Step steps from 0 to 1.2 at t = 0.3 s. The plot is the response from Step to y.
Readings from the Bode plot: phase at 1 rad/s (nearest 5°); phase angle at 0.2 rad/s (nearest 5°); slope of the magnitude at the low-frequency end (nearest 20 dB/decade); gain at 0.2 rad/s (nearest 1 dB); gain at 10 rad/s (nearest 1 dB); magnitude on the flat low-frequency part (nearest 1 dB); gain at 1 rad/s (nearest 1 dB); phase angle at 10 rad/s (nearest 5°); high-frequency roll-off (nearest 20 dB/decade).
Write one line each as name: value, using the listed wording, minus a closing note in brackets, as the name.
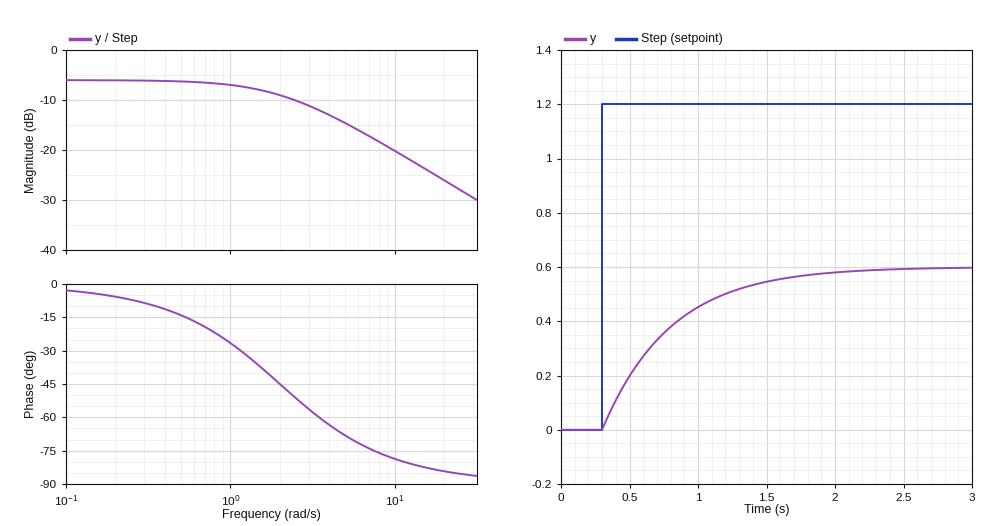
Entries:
phase at 1 rad/s: -25°
phase angle at 0.2 rad/s: -5°
slope of the magnitude at the low-frequency end: 0 dB/decade
gain at 0.2 rad/s: -6 dB
gain at 10 rad/s: -20 dB
magnitude on the flat low-frequency part: -6 dB
gain at 1 rad/s: -7 dB
phase angle at 10 rad/s: -80°
high-frequency roll-off: -20 dB/decade
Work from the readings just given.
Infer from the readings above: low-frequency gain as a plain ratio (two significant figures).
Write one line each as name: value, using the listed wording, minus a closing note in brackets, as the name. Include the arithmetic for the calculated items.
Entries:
low-frequency gain as a plain ratio: 10^(-6 / 20) = 0.50
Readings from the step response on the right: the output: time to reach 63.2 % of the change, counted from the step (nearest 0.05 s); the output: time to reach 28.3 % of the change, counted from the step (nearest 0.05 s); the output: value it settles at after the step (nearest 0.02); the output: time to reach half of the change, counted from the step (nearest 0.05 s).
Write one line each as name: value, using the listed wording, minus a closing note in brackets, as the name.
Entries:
the output: time to reach 63.2 % of the change, counted from the step: 0.50 s
the output: time to reach 28.3 % of the change, counted from the step: 0.15 s
the output: value it settles at after the step: 0.60
the output: time to reach half of the change, counted from the step: 0.35 s
